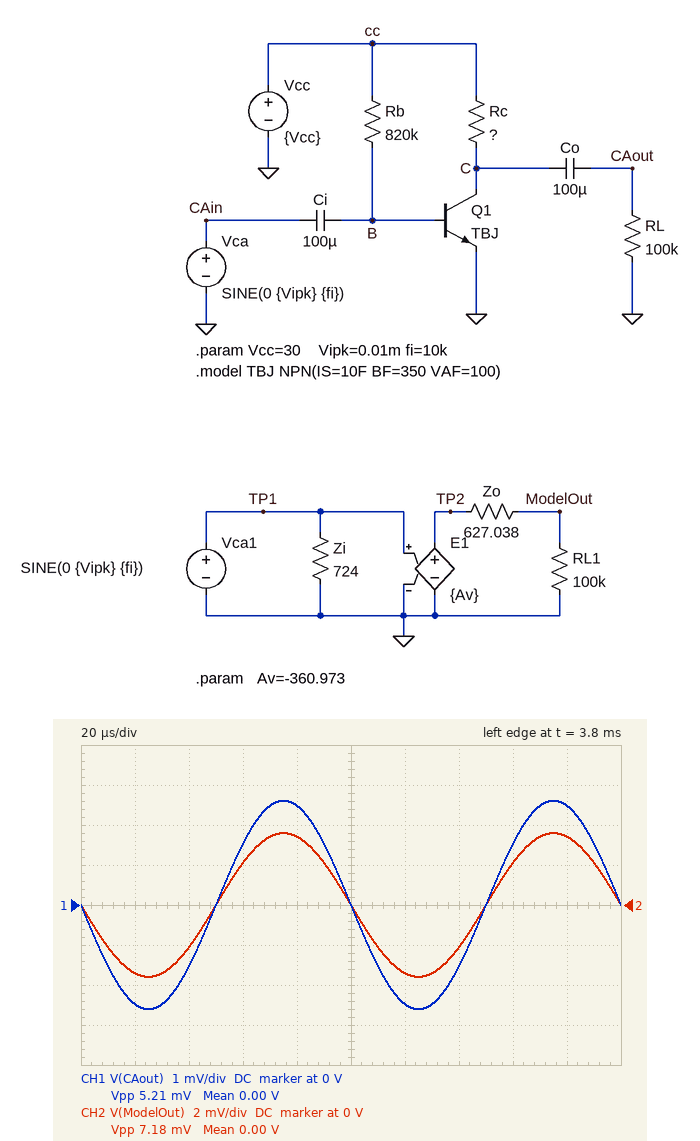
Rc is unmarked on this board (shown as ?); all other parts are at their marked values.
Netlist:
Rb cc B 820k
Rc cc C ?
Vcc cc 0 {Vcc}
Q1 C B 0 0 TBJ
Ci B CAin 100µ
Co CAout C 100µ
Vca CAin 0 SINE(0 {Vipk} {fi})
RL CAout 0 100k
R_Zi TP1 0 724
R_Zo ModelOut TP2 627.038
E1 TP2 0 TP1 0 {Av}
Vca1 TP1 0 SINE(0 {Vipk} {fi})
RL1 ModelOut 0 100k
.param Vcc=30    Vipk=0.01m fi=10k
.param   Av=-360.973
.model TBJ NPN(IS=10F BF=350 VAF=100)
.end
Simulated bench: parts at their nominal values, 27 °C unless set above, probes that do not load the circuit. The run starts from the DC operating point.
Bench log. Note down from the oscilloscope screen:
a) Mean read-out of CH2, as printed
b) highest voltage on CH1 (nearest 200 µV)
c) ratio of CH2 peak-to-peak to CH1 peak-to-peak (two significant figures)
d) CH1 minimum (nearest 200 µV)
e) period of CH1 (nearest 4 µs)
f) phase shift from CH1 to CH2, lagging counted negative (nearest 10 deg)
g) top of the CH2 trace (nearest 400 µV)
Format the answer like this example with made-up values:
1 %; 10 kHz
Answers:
0.00 V; 2.6 mV; 1.4; -2.6 mV; 100 µs; 0 deg; 3.6 mV
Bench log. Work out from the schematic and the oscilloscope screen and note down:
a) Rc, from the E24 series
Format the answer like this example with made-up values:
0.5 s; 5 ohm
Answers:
470 Ω
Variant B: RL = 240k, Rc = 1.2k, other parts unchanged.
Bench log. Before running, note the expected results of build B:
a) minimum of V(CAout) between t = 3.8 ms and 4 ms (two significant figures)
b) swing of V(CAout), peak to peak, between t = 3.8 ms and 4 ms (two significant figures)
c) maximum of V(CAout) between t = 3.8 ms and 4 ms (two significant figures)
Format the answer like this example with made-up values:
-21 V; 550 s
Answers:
-5.6 mV; 11 mV; 5.6 mV
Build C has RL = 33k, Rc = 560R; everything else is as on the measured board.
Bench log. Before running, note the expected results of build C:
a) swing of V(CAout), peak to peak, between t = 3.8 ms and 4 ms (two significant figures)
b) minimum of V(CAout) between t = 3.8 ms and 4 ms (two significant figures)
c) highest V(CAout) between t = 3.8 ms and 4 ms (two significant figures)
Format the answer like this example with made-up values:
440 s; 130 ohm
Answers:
6.0 mV; -3.0 mV; 3.0 mV
